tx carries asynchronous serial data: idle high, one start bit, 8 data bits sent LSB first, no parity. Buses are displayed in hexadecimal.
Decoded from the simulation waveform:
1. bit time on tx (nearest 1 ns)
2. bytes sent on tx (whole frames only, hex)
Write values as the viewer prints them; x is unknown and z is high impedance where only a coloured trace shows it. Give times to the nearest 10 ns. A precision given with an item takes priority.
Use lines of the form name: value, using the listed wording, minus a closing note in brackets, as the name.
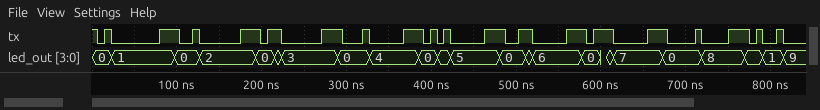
bit time on tx: 8 ns
bytes sent on tx: 01, 02, 03, 04, 05, 06, 07, 08
